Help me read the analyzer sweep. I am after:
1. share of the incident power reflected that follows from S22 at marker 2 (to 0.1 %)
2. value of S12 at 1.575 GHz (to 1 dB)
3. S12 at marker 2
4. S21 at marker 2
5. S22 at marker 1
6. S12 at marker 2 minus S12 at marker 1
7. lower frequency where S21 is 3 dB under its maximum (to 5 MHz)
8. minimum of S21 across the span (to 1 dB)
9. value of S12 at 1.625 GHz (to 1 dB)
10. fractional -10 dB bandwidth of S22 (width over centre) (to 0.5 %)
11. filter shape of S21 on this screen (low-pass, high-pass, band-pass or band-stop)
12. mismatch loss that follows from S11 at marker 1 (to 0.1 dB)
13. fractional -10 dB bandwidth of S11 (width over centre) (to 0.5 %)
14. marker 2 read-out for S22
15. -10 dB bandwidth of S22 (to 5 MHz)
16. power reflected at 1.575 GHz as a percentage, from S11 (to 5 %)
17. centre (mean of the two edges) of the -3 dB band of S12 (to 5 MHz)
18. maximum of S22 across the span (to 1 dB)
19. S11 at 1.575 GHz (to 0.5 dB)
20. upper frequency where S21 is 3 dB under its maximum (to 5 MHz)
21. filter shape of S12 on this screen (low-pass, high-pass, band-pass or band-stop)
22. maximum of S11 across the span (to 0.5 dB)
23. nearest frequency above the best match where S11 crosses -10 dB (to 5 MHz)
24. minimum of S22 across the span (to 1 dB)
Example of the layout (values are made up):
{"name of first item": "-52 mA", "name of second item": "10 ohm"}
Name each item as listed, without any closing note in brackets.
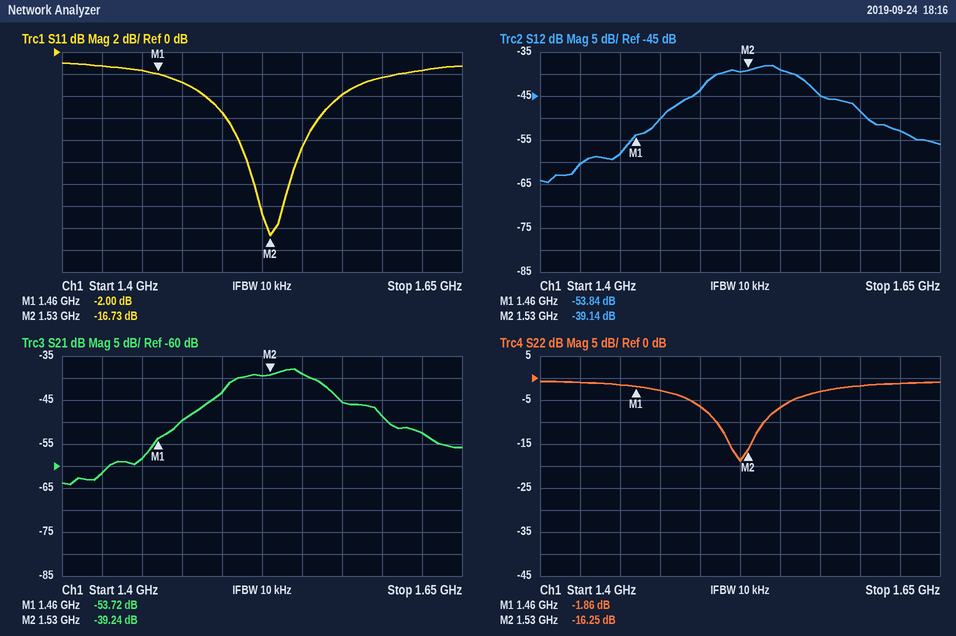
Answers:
{"share of the incident power reflected that follows from S22 at marker 2": "2.4 %", "value of S12 at 1.575 GHz": "-45 dB", "S12 at marker 2": "-39.14 dB", "S21 at marker 2": "-39.24 dB", "S22 at marker 1": "-1.86 dB", "S12 at marker 2 minus S12 at marker 1": "14.70 dB", "lower frequency where S21 is 3 dB under its maximum": "1.505 GHz", "minimum of S21 across the span": "-64 dB", "value of S12 at 1.625 GHz": "-53 dB", "fractional -10 dB bandwidth of S22 (width over centre)": "2.0 %", "filter shape of S21 on this screen": "band-pass", "mismatch loss that follows from S11 at marker 1": "4.3 dB", "fractional -10 dB bandwidth of S11 (width over centre)": "2.0 %", "marker 2 read-out for S22": "-16.25 dB", "-10 dB bandwidth of S22": "30 MHz", "power reflected at 1.575 GHz as a percentage, from S11": "40 %", "centre (mean of the two edges) of the -3 dB band of S12": "1.535 GHz", "maximum of S22 across the span": "-1 dB", "S11 at 1.575 GHz": "-4.0 dB", "upper frequency where S21 is 3 dB under its maximum": "1.560 GHz", "filter shape of S12 on this screen": "band-pass", "maximum of S11 across the span": "-1.0 dB", "nearest frequency above the best match where S11 crosses -10 dB": "1.545 GHz", "minimum of S22 across the span": "-19 dB"}
